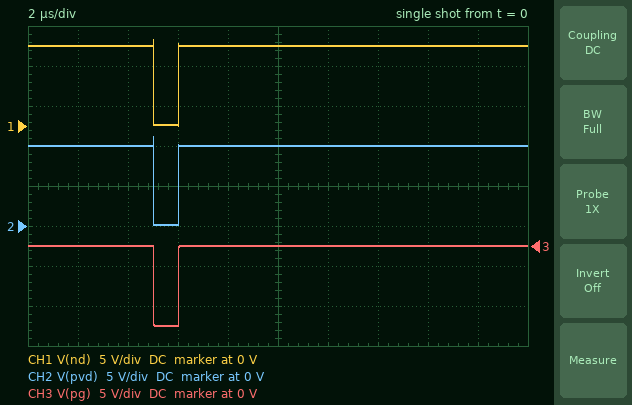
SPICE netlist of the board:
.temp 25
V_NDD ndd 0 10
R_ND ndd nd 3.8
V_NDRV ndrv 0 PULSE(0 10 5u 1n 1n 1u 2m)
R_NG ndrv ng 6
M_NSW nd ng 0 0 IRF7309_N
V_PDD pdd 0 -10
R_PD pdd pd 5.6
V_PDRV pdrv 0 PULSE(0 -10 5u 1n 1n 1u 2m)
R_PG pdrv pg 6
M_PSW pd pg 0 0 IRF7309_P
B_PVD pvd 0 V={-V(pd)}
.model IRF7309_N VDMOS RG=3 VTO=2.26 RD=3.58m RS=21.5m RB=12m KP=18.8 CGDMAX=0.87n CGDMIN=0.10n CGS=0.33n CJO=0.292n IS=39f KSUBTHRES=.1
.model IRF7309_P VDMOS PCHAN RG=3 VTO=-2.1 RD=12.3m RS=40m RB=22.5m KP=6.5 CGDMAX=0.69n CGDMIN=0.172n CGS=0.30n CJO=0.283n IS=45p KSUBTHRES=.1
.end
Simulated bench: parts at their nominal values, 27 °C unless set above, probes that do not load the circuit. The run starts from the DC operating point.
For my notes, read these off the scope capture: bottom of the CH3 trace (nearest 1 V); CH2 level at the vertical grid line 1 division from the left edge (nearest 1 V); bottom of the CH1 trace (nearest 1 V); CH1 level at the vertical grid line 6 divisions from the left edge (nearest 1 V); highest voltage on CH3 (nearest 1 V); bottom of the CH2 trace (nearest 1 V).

-10 V
10 V
0 V
10 V
0 V
0 V
